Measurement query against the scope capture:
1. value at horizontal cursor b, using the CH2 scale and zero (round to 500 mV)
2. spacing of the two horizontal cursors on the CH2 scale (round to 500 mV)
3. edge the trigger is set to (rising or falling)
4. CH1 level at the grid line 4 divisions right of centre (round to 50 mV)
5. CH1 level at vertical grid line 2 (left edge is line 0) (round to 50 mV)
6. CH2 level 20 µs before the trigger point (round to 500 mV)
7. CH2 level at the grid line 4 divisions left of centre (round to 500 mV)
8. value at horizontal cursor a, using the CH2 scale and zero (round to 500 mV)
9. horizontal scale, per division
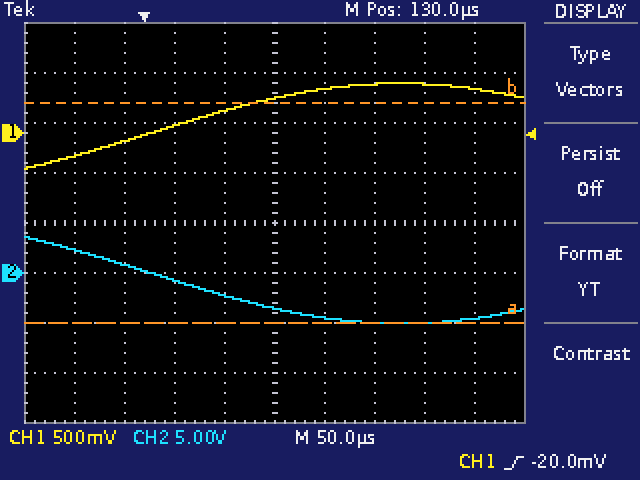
17.0 V
22.0 V
rising
450 mV
-100 mV
1.0 V
2.5 V
-5.0 V
50 µs
